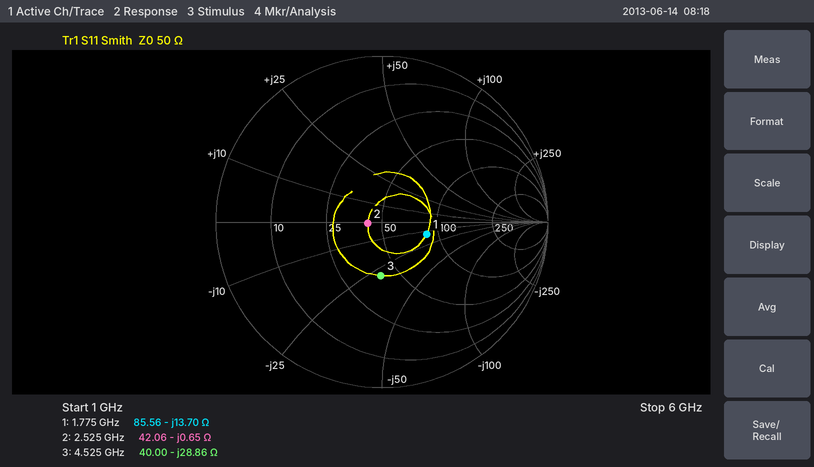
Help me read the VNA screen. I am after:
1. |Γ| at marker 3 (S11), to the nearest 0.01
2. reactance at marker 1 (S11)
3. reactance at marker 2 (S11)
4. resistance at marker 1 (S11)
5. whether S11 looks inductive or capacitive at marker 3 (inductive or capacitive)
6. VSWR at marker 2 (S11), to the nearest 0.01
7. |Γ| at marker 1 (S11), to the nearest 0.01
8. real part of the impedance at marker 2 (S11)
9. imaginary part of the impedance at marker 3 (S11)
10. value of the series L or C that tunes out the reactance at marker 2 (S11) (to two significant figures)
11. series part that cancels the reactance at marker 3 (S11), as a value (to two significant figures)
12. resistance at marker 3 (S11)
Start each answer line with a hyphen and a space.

- 0.32
- -13.70 Ω
- -0.65 Ω
- 85.56 Ω
- capacitive
- 1.19
- 0.28
- 42.06 Ω
- -28.86 Ω
- 41 pH
- 1.0 nH
- 40.00 Ω
